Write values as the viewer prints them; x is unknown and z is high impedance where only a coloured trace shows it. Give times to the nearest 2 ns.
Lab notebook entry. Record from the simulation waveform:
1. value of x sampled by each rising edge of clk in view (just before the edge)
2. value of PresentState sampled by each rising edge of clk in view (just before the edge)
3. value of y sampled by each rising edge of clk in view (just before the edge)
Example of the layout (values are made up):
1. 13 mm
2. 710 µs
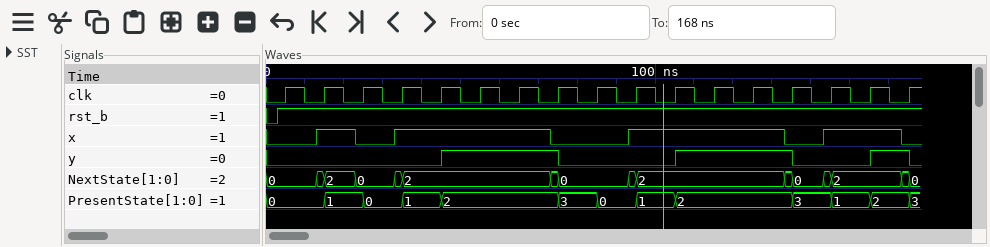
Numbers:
1. 0 1 0 1 1 1 1 0 0 1 1 1 1 0 1 1 0
2. 0, 0, 1, 0, 1, 2, 2, 2, 3, 0, 1, 2, 2, 2, 3, 1, 2
3. 0 0 0 0 0 1 1 1 0 0 0 1 1 1 0 0 1
